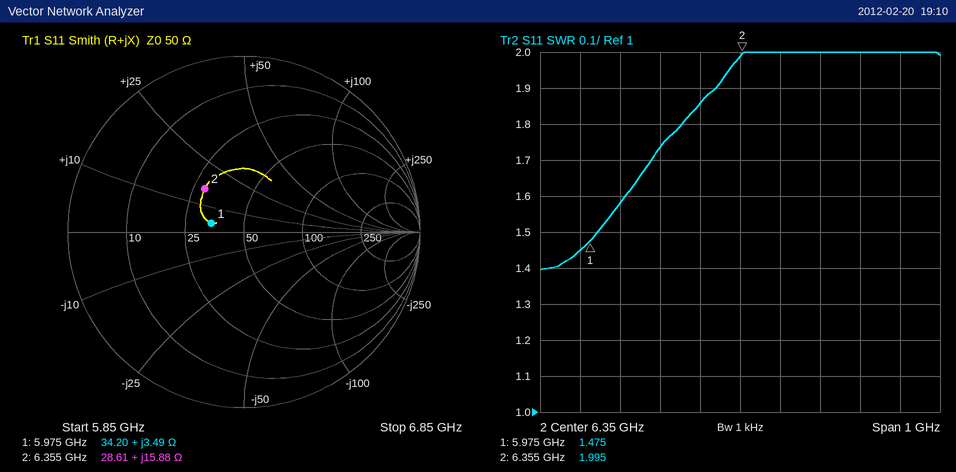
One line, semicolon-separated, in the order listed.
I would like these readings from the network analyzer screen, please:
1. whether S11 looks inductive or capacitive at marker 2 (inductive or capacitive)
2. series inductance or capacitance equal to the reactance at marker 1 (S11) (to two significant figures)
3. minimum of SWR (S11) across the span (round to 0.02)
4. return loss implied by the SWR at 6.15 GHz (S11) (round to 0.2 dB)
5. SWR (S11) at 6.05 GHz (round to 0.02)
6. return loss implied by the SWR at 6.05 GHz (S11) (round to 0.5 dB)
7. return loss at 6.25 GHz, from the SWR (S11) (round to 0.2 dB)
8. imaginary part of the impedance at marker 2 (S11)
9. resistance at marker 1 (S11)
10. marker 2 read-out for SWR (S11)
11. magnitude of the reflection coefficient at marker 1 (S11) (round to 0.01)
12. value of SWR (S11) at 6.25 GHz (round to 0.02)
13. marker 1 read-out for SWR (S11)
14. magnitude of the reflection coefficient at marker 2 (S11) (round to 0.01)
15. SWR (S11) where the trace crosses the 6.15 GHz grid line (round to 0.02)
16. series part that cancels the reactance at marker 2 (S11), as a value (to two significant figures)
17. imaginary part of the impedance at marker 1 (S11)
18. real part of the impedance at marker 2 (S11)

inductive; 93 pH; 1.40; 11.4 dB; 1.58; 13.0 dB; 10.4 dB; +15.88 Ω; 34.20 Ω; 1.995; 0.19; 1.86; 1.475; 0.33; 1.74; 1.6 pF; +3.49 Ω; 28.61 Ω
